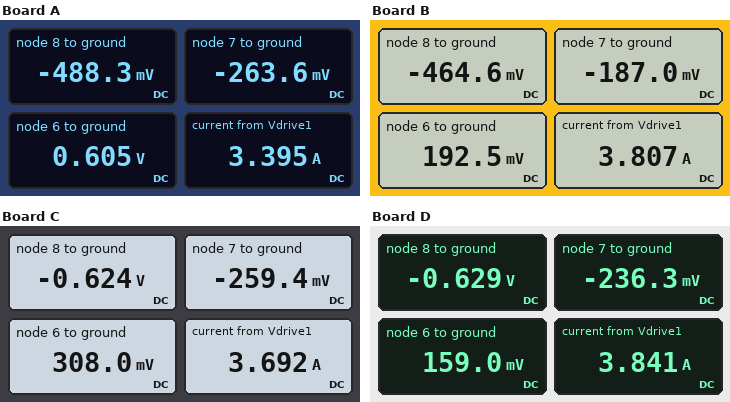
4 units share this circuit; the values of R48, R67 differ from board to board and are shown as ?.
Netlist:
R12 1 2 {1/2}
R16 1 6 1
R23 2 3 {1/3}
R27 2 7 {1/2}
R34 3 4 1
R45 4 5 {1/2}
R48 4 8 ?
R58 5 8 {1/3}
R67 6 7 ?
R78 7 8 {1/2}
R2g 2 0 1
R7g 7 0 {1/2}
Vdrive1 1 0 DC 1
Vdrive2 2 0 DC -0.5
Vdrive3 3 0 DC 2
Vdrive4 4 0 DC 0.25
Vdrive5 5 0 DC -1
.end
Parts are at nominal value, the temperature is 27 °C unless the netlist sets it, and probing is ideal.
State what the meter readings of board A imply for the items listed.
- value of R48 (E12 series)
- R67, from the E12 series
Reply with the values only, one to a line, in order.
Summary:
0.68 Ω
2.2 Ω
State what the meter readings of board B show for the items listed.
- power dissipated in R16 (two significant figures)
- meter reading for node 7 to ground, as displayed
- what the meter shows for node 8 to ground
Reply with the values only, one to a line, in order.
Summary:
650 mW
-187.0 mV
-464.6 mV
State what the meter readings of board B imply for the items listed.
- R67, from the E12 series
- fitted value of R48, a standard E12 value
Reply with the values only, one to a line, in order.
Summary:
0.47 Ω
0.68 Ω
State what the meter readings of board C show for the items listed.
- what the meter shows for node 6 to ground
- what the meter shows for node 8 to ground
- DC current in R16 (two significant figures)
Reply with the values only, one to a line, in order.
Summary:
308.0 mV
-0.624 V
690 mA
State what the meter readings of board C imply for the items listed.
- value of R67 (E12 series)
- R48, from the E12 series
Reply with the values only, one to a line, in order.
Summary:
0.82 Ω
2.2 Ω
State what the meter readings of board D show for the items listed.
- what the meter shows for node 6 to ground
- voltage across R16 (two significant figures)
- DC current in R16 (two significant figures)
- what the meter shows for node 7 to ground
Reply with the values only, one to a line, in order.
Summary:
159.0 mV
840 mV
840 mA
-236.3 mV
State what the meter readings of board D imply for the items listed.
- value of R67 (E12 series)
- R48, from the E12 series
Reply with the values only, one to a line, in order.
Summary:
0.47 Ω
2.7 Ω
